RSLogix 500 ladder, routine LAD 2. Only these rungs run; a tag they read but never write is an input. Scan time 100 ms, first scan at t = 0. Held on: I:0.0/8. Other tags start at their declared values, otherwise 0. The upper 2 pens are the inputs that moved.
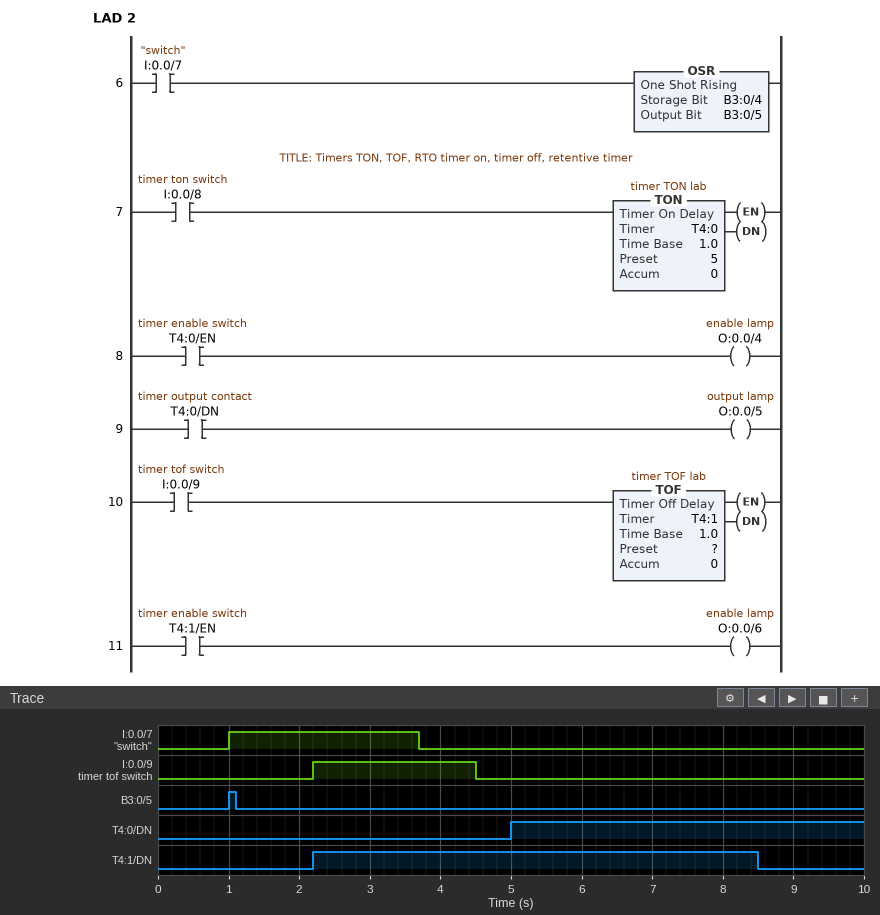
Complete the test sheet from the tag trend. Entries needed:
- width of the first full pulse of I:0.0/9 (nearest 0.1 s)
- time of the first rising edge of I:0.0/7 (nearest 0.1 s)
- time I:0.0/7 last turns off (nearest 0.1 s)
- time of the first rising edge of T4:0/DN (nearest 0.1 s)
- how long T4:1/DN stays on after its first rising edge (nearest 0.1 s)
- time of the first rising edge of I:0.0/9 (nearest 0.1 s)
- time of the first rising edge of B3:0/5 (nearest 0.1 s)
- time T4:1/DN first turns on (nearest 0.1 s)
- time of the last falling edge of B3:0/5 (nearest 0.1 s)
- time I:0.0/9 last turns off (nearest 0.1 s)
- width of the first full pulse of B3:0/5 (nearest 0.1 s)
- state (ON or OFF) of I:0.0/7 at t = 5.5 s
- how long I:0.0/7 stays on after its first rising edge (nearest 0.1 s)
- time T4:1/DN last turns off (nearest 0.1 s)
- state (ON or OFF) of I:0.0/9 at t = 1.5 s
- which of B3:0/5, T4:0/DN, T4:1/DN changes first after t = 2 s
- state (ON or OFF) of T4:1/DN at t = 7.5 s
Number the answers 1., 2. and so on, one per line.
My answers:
1. 2.3 s
2. 1.0 s
3. 3.7 s
4. 5.0 s
5. 6.3 s
6. 2.2 s
7. 1.0 s
8. 2.2 s
9. 1.1 s
10. 4.5 s
11. 0.1 s
12. OFF
13. 2.7 s
14. 8.5 s
15. OFF
16. T4:1/DN
17. ON
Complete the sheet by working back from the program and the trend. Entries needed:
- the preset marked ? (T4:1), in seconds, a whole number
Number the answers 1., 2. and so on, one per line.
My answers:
1. 4 s
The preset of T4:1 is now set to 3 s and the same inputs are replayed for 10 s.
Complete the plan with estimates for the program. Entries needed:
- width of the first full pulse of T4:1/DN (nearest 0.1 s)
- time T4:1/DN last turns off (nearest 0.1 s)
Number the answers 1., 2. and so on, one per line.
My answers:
1. 5.3 s
2. 7.5 s
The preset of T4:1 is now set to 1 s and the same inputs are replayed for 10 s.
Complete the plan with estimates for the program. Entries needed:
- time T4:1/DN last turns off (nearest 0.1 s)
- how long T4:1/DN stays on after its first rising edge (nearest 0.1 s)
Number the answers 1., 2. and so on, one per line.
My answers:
1. 5.5 s
2. 3.3 s
